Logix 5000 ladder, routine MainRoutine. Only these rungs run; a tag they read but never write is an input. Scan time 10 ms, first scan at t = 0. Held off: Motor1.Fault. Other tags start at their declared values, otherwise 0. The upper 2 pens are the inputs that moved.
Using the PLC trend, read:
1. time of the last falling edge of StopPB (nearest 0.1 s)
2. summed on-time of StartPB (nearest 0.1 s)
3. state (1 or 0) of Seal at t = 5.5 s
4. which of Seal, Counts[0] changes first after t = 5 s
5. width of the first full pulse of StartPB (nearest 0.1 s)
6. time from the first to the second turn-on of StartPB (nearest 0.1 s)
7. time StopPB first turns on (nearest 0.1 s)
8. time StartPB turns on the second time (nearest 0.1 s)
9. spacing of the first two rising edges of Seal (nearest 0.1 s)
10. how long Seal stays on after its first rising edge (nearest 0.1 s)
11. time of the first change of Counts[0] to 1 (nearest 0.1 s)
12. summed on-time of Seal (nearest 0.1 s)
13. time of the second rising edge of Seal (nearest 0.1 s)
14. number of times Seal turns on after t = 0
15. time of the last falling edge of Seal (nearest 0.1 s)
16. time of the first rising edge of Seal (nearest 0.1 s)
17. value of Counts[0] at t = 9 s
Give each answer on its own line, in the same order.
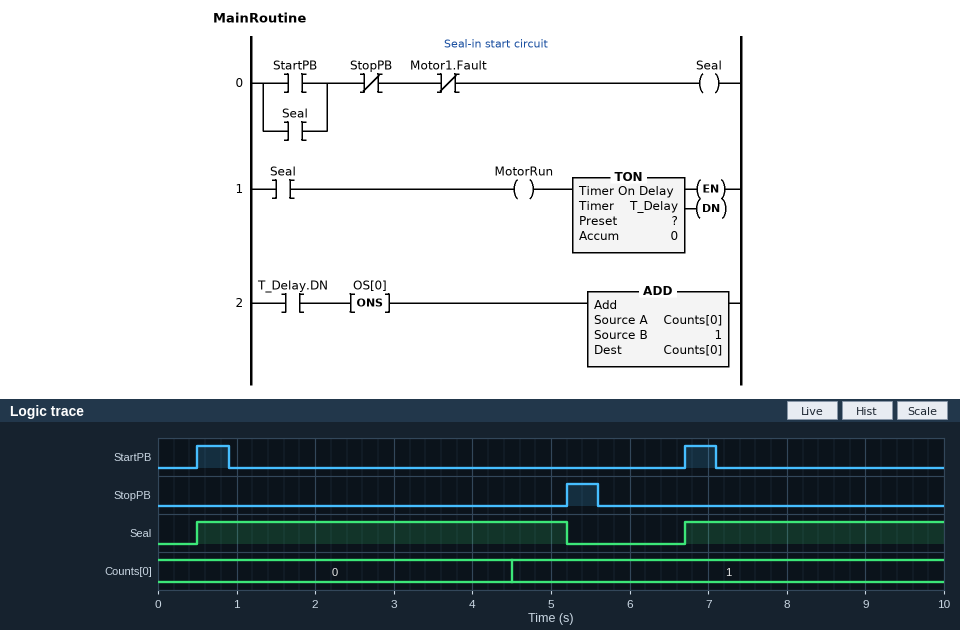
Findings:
5.6 s
0.8 s
0
Seal
0.4 s
6.2 s
5.2 s
6.7 s
6.2 s
4.7 s
4.5 s
8.0 s
6.7 s
2
5.2 s
0.5 s
1
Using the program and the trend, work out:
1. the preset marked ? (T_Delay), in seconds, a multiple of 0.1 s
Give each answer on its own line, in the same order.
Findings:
4.0 s
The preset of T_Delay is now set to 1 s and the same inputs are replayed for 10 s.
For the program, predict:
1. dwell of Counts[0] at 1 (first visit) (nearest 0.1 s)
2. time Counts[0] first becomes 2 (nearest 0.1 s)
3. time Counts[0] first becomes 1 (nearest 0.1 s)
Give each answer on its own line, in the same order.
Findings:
6.2 s
7.7 s
1.5 s
